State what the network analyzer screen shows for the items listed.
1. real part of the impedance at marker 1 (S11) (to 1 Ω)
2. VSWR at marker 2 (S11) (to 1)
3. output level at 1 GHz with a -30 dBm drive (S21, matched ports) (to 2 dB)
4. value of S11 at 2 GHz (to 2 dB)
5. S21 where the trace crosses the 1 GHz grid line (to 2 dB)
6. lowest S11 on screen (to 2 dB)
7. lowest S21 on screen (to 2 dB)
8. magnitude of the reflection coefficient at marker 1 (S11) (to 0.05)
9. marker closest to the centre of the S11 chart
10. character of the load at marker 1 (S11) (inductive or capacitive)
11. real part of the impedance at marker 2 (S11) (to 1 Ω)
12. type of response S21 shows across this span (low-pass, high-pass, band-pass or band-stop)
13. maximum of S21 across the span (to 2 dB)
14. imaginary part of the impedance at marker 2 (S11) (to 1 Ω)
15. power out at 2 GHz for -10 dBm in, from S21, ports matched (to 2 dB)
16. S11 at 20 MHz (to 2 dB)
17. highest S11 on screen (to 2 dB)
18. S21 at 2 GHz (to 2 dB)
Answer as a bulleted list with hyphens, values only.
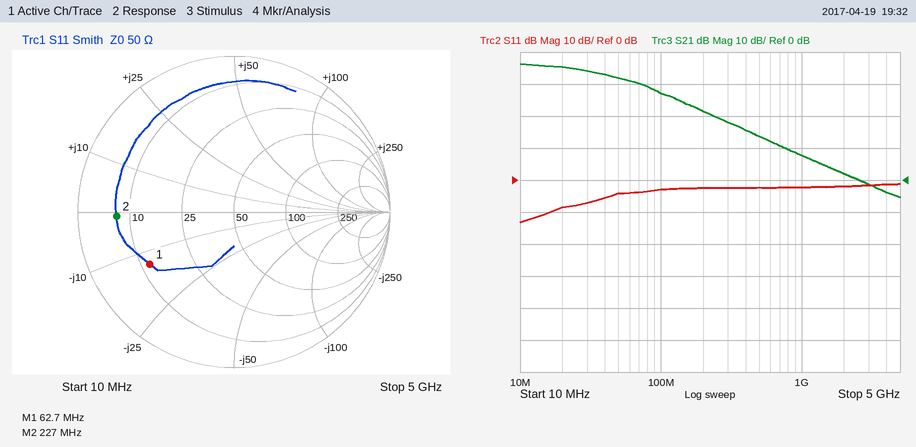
- 12 Ω
- 7
- -22 dBm
- -2 dB
- 8 dB
- -14 dB
- -6 dB
- 0.65
- marker 1
- capacitive
- 7 Ω
- low-pass
- 36 dB
- -1 Ω
- -8 dBm
- -8 dB
- -2 dB
- 2 dB
